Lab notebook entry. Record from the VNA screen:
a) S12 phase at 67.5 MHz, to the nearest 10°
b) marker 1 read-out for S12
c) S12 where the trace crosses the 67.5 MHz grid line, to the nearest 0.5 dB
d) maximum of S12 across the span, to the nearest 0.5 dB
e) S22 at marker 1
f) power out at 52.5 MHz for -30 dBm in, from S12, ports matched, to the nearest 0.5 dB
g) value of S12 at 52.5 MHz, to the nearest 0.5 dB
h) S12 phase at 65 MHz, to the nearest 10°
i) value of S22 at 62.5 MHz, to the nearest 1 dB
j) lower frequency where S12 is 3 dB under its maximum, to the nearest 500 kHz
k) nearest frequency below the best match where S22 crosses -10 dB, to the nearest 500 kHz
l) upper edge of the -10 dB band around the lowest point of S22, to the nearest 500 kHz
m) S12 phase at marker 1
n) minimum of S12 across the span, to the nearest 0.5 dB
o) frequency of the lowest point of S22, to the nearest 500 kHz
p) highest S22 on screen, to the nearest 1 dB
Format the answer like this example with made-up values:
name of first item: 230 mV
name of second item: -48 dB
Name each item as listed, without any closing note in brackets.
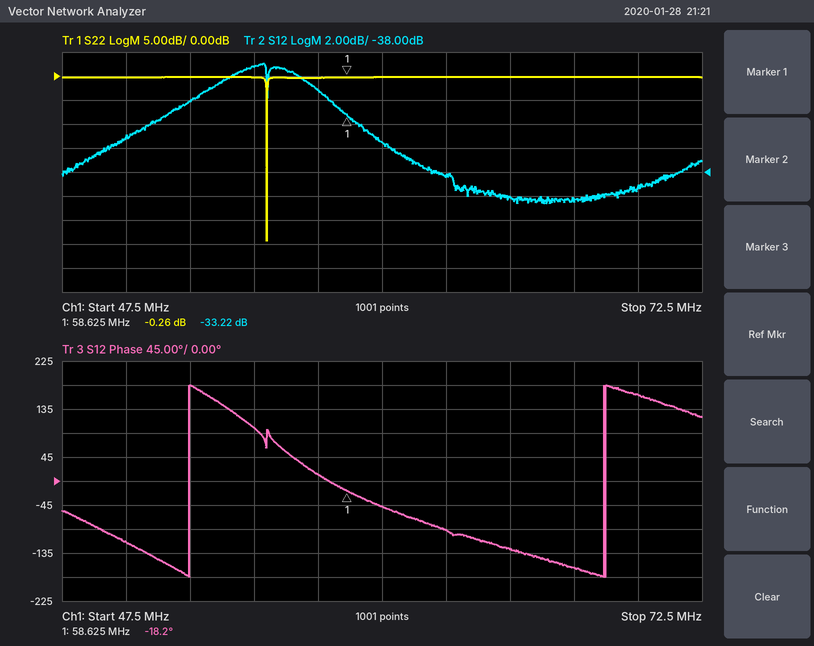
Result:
S12 phase at 67.5 MHz, to the nearest 10°: -160°
marker 1 read-out for S12: -33.22 dB
S12 where the trace crosses the 67.5 MHz grid line, to the nearest 0.5 dB: -40.5 dB
maximum of S12 across the span, to the nearest 0.5 dB: -29.0 dB
S22 at marker 1: -0.26 dB
power out at 52.5 MHz for -30 dBm in, from S12, ports matched, to the nearest 0.5 dB: -62.0 dBm
value of S12 at 52.5 MHz, to the nearest 0.5 dB: -32.0 dB
S12 phase at 65 MHz, to the nearest 10°: -130°
value of S22 at 62.5 MHz, to the nearest 1 dB: 0 dB
lower frequency where S12 is 3 dB under its maximum, to the nearest 500 kHz: 52.5 MHz
nearest frequency below the best match where S22 crosses -10 dB, to the nearest 500 kHz: 55.5 MHz
upper edge of the -10 dB band around the lowest point of S22, to the nearest 500 kHz: 55.5 MHz
S12 phase at marker 1: -18.2°
minimum of S12 across the span, to the nearest 0.5 dB: -40.5 dB
frequency of the lowest point of S22, to the nearest 500 kHz: 55.5 MHz
highest S22 on screen, to the nearest 1 dB: 0 dB
